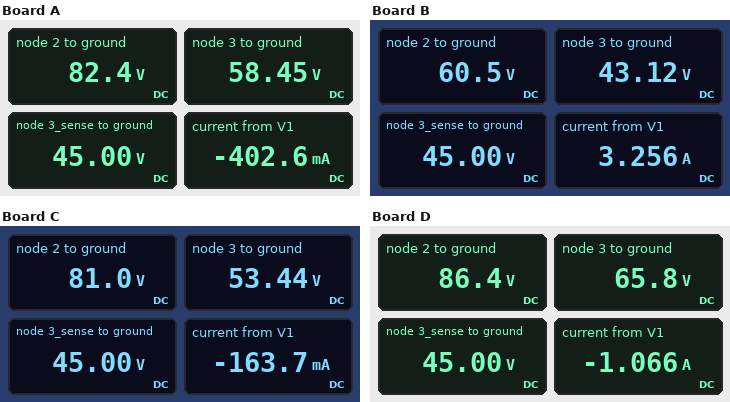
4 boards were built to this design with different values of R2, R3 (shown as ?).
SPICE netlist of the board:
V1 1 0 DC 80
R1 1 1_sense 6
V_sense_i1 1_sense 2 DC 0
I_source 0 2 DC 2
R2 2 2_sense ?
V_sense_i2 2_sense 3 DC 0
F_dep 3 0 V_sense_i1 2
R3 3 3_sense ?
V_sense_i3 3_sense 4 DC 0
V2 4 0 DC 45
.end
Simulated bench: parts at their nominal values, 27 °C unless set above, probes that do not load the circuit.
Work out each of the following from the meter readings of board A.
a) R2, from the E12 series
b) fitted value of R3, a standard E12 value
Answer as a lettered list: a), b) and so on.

a) 15 Ω
b) 5.6 Ω
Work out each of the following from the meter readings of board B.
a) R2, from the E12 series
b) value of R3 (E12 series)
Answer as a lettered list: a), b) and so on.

a) 3.3 Ω
b) 1.5 Ω
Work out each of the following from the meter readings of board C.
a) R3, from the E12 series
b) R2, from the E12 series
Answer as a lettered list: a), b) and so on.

a) 3.9 Ω
b) 15 Ω
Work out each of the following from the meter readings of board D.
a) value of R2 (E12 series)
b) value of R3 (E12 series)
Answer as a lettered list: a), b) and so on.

a) 22 Ω
b) 6.8 Ω
